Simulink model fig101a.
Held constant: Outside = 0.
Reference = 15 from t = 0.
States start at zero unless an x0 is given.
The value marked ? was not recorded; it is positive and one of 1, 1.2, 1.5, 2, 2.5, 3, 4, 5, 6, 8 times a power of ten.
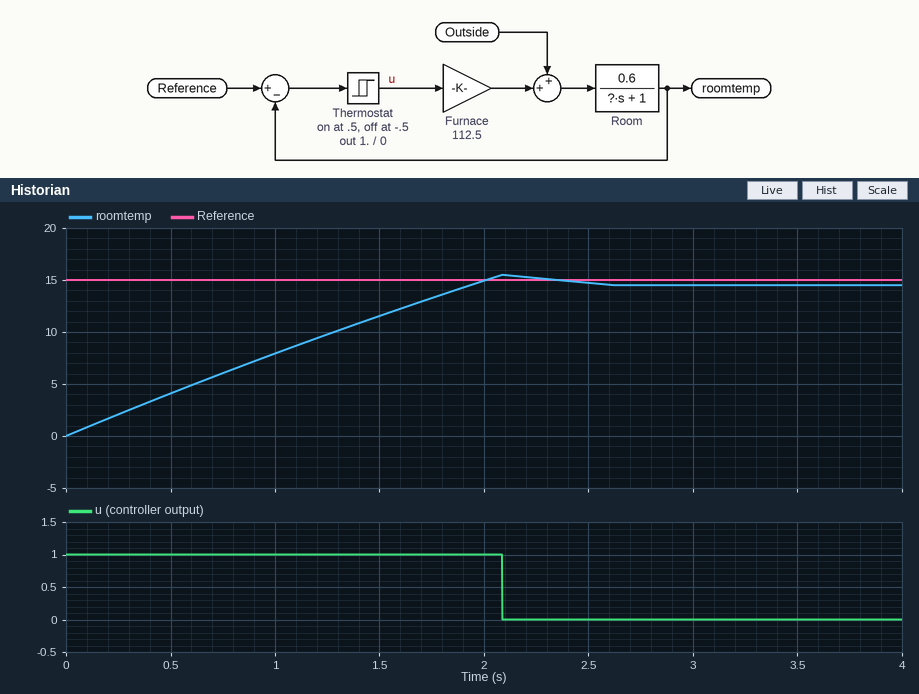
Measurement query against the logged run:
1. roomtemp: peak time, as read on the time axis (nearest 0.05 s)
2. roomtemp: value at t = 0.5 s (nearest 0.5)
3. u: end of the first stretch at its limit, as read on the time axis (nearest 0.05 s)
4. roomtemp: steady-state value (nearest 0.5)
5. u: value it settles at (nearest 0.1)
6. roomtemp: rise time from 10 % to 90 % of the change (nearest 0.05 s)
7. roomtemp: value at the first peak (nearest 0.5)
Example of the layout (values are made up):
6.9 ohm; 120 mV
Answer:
2.10 s; 4.0; 2.10 s; 14.5; 0.0; 1.55 s; 15.5
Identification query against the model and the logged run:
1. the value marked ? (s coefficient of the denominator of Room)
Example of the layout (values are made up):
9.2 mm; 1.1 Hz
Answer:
8
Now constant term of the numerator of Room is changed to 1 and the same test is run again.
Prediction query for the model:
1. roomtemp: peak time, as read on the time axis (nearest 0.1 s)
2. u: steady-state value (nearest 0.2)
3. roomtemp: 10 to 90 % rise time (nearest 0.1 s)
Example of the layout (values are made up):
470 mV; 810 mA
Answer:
1.2 s; 0.0; 0.9 s
